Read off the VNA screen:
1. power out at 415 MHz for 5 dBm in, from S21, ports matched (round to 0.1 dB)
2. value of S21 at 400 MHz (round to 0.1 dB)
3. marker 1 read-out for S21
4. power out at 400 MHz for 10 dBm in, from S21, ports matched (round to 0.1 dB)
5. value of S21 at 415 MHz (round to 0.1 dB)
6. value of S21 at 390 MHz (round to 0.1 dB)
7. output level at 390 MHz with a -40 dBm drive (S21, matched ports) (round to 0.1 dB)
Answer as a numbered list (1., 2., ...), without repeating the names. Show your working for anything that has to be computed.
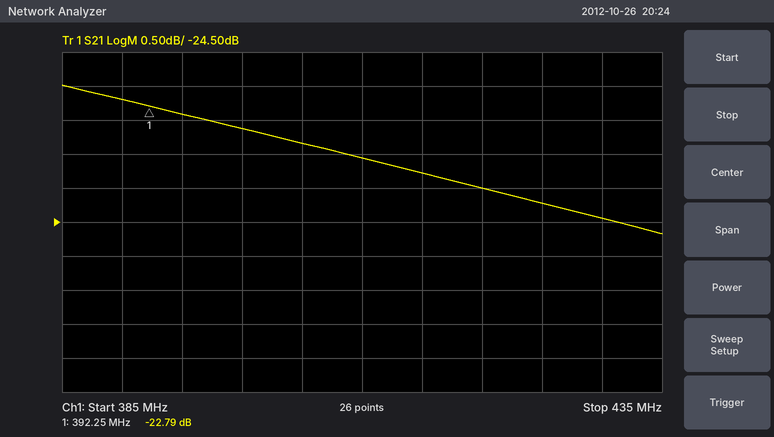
1. 5 dBm + (-23.8 dB) = -18.8 dBm
2. -23.1 dB
3. -22.79 dB
4. 10 dBm + (-23.1 dB) = -13.1 dBm
5. -23.8 dB
6. -22.7 dB
7. -40 dBm + (-22.7 dB) = -62.7 dBm
